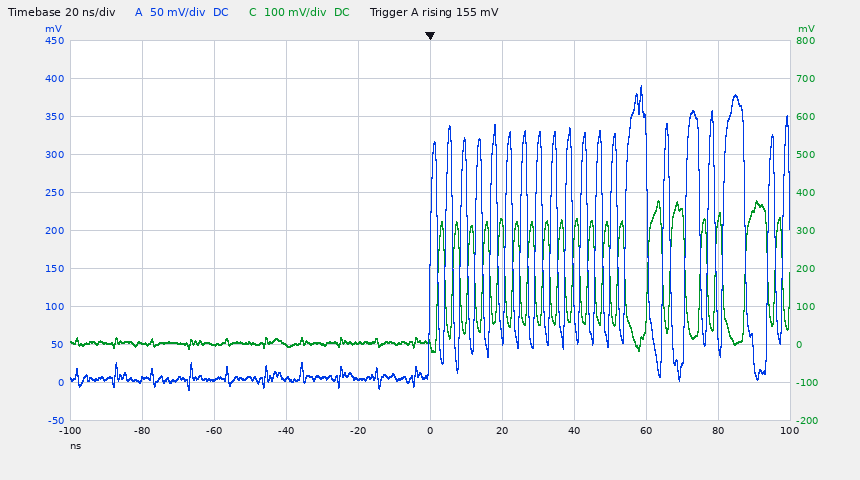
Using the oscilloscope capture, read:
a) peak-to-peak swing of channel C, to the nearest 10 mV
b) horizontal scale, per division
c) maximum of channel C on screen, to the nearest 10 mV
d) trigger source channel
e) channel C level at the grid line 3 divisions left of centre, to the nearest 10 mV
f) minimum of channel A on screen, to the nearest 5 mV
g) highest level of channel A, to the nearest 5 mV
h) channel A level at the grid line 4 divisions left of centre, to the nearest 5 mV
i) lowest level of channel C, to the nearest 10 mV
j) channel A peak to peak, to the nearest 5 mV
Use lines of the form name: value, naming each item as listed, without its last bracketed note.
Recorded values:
peak-to-peak swing of channel C, to the nearest 10 mV: 400 mV
horizontal scale, per division: 20 ns
maximum of channel C on screen, to the nearest 10 mV: 380 mV
trigger source channel: channel A
channel C level at the grid line 3 divisions left of centre, to the nearest 10 mV: 0 mV
minimum of channel A on screen, to the nearest 5 mV: -10 mV
highest level of channel A, to the nearest 5 mV: 390 mV
channel A level at the grid line 4 divisions left of centre, to the nearest 5 mV: 5 mV
lowest level of channel C, to the nearest 10 mV: -20 mV
channel A peak to peak, to the nearest 5 mV: 400 mV
